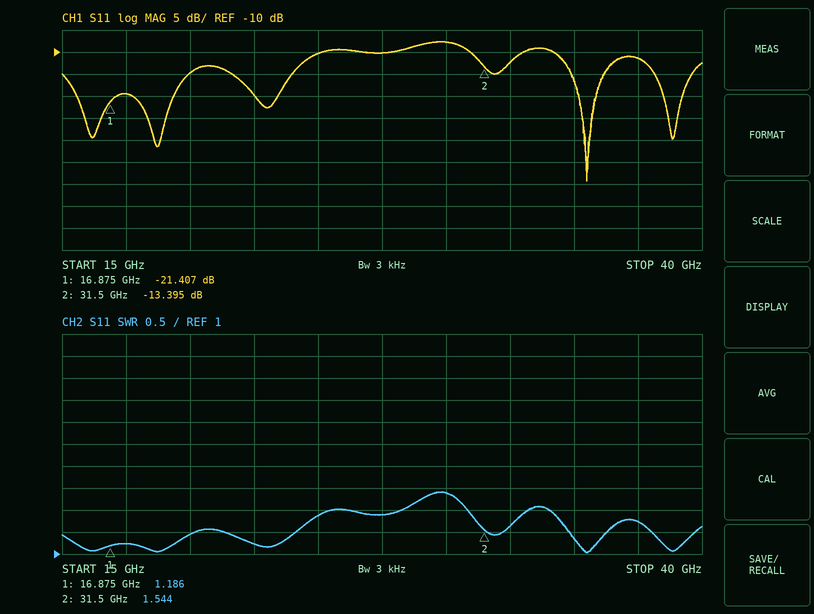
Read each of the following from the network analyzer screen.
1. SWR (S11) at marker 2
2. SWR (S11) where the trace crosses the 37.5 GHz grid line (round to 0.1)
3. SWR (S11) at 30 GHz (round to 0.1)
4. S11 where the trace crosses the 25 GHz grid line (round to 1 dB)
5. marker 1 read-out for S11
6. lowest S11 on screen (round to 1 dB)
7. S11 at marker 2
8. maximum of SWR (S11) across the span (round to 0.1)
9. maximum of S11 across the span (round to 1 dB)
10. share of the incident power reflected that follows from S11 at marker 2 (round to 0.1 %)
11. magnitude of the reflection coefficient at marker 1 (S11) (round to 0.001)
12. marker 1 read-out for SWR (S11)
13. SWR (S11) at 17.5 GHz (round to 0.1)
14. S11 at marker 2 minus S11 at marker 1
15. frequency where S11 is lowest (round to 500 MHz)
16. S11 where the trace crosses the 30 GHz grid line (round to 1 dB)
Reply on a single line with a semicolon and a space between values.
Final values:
1.544; 1.7; 2.4; -10 dB; -21.407 dB; -39 dB; -13.395 dB; 2.4; -8 dB; 4.6 %; 0.085; 1.186; 1.2; 8.012 dB; 35.5 GHz; -8 dB
